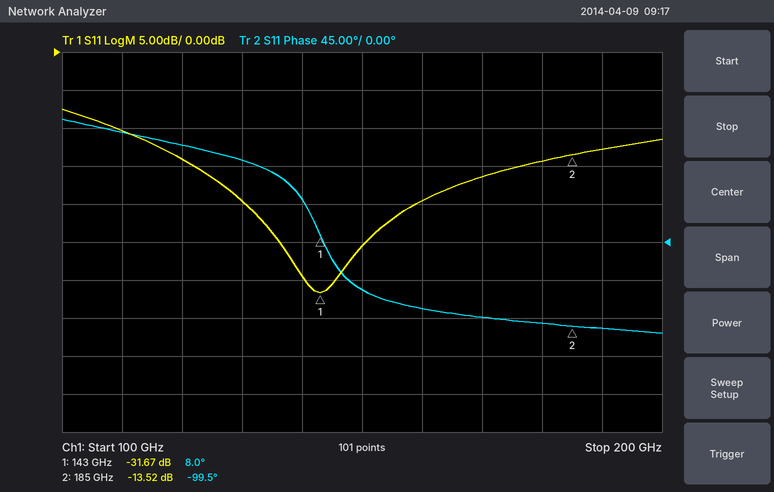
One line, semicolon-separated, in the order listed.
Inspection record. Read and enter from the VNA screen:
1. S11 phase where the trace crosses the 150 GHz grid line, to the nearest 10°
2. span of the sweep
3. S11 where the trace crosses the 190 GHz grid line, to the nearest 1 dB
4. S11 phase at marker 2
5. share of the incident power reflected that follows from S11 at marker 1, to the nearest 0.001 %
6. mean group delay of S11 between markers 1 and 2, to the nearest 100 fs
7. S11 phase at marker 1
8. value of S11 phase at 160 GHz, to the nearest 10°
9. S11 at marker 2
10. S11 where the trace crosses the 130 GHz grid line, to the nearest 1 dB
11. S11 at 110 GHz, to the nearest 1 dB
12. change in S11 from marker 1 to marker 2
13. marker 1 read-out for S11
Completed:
-60°; 100 GHz; -13 dB; -99.5°; 0.068 %; 7.1 ps; 8.0°; -80°; -13.52 dB; -20 dB; -10 dB; 18.15 dB; -31.67 dB
